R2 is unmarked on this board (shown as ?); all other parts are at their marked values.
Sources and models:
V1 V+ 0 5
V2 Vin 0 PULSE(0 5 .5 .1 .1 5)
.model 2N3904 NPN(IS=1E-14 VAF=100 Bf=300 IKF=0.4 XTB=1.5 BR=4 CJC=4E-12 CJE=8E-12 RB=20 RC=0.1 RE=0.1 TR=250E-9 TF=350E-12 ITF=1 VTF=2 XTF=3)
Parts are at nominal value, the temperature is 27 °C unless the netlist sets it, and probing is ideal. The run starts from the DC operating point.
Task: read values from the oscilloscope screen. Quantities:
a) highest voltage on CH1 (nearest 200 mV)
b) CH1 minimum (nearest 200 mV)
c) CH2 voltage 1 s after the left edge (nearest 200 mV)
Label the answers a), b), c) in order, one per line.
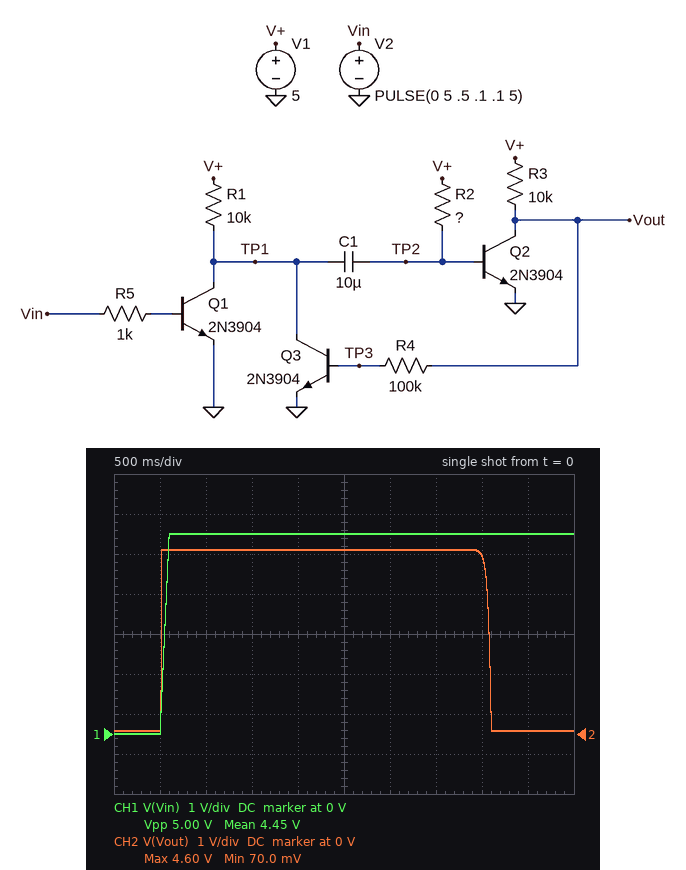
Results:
a) 5.0 V
b) 0 V
c) 4.6 V
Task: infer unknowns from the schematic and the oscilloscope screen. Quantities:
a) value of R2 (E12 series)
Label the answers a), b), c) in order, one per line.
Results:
a) 470 kΩ
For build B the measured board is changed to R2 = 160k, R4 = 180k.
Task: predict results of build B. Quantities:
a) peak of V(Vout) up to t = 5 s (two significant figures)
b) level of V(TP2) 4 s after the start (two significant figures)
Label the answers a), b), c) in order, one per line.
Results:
a) 4.8 V
b) 640 mV
